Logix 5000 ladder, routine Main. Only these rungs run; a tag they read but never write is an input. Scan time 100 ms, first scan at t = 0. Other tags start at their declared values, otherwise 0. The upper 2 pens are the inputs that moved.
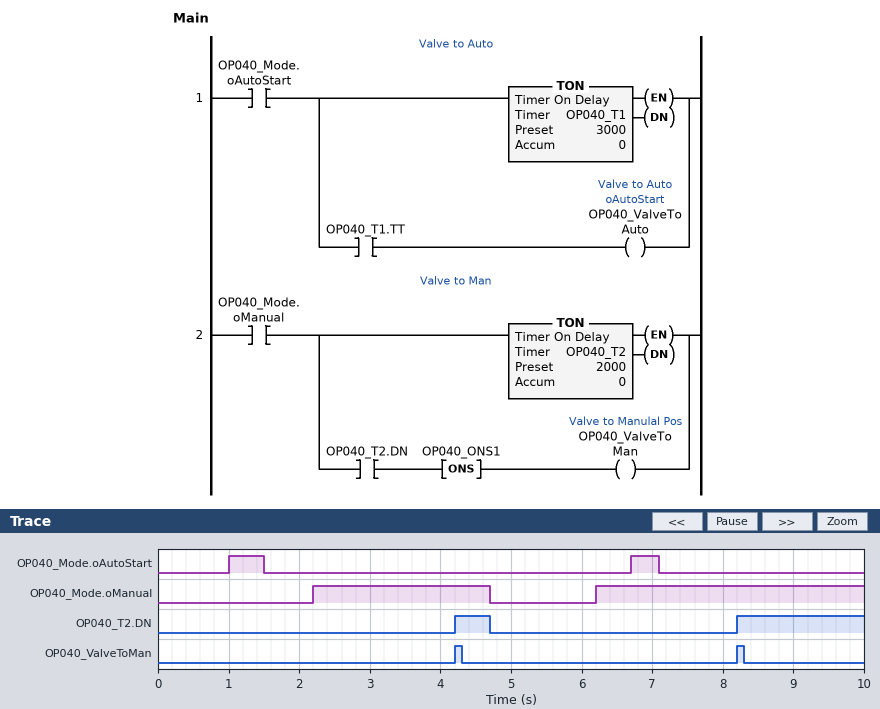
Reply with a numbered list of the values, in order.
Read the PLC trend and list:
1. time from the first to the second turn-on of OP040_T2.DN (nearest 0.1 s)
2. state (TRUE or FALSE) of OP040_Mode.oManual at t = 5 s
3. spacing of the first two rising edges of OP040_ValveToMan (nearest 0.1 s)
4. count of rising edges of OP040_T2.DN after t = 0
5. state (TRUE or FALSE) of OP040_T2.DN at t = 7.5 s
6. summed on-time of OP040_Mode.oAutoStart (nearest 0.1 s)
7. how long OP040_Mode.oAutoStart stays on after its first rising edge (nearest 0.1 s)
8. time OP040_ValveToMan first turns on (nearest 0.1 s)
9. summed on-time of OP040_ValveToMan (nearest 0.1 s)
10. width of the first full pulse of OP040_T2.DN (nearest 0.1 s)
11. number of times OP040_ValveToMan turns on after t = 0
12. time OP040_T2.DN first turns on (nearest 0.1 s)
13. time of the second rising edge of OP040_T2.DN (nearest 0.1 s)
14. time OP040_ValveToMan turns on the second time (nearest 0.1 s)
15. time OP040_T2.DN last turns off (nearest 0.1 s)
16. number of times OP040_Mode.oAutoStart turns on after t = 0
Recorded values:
1. 4.0 s
2. FALSE
3. 4.0 s
4. 2
5. FALSE
6. 0.9 s
7. 0.5 s
8. 4.2 s
9. 0.2 s
10. 0.5 s
11. 2
12. 4.2 s
13. 8.2 s
14. 8.2 s
15. 4.7 s
16. 2
